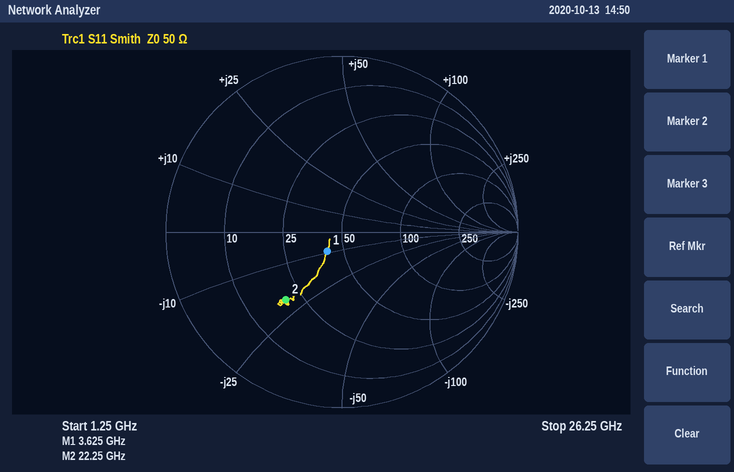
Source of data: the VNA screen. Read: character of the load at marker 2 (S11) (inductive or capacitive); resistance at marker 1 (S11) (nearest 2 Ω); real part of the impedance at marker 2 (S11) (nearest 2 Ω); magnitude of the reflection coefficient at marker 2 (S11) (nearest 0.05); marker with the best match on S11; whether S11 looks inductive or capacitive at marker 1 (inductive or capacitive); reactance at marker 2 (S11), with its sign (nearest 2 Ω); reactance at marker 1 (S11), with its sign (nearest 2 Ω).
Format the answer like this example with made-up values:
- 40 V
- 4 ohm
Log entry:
- capacitive
- 42 Ω
- 20 Ω
- 0.50
- marker 1
- capacitive
- -20 Ω
- -10 Ω
